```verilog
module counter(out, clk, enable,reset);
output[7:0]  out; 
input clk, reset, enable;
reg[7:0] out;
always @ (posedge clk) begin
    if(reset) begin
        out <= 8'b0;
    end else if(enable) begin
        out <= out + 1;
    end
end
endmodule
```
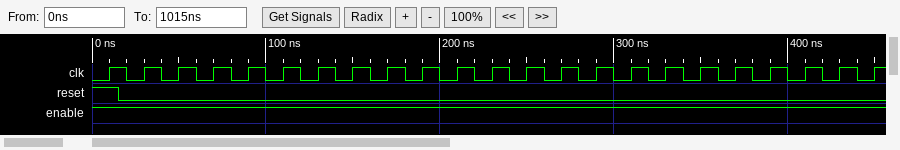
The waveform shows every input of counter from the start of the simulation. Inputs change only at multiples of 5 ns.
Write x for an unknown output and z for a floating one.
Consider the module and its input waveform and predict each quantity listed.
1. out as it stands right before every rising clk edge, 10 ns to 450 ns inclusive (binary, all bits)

x, 00000000, 00000001, 00000010, 00000011, 00000100, 00000101, 00000110, 00000111, 00001000, 00001001, 00001010, 00001011, 00001100, 00001101, 00001110, 00001111, 00010000, 00010001, 00010010, 00010011, 00010100, 00010101
